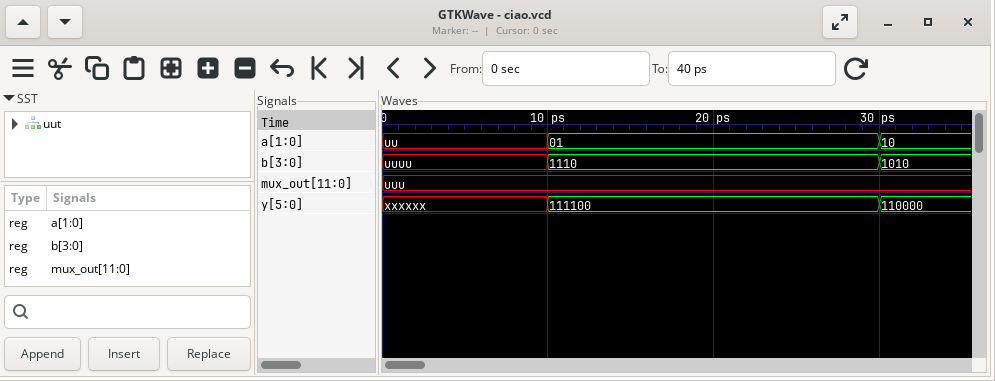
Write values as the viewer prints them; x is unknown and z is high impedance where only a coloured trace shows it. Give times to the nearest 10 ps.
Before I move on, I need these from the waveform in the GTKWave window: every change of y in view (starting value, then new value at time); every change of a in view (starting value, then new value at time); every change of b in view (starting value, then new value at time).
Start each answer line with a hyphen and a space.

- xxxxxx, 111100 at 10 ps, 110000 at 30 ps
- uu, 01 at 10 ps, 10 at 30 ps
- uuuu, 1110 at 10 ps, 1010 at 30 ps
